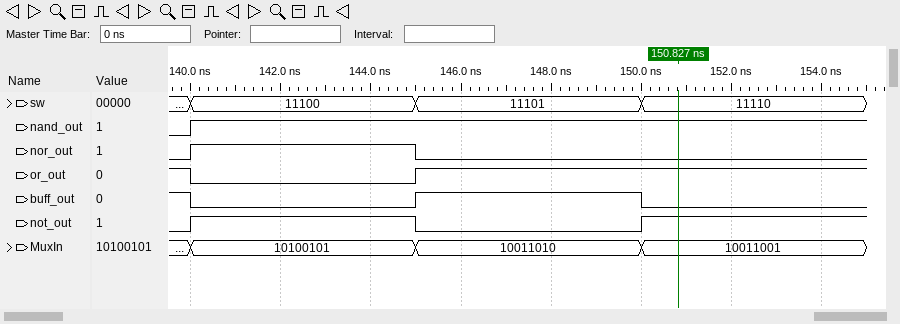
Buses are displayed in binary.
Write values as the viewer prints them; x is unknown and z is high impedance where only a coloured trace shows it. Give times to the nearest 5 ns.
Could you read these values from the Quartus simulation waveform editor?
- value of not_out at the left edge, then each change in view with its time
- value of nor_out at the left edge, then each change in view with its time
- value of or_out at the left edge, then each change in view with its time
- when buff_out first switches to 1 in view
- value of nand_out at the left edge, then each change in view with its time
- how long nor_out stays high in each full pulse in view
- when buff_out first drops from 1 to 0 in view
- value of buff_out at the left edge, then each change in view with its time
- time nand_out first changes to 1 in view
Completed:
0, 1 at 140 ns, 0 at 145 ns, 1 at 150 ns
0, 1 at 140 ns, 0 at 145 ns
1, 0 at 140 ns, 1 at 145 ns
145 ns
0, 1 at 140 ns
5 ns
140 ns
1, 0 at 140 ns, 1 at 145 ns, 0 at 150 ns
140 ns
